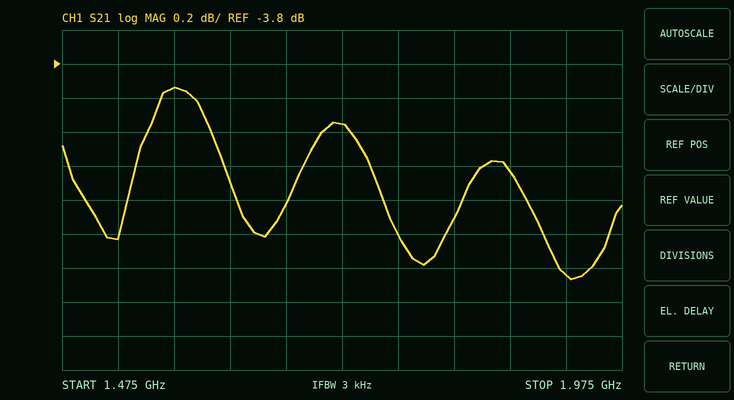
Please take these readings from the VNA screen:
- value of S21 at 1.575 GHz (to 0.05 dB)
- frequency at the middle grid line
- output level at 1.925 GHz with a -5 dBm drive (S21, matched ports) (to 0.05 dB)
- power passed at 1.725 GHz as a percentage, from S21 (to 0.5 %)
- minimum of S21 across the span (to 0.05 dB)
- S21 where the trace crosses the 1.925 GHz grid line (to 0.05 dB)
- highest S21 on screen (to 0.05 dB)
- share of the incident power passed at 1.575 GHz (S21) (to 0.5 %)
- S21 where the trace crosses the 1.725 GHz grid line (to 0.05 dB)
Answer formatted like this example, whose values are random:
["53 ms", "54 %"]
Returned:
["-3.95 dB", "1.725 GHz", "-10.05 dBm", "38.5 %", "-5.05 dB", "-5.05 dB", "-3.95 dB", "40.5 %", "-4.15 dB"]
